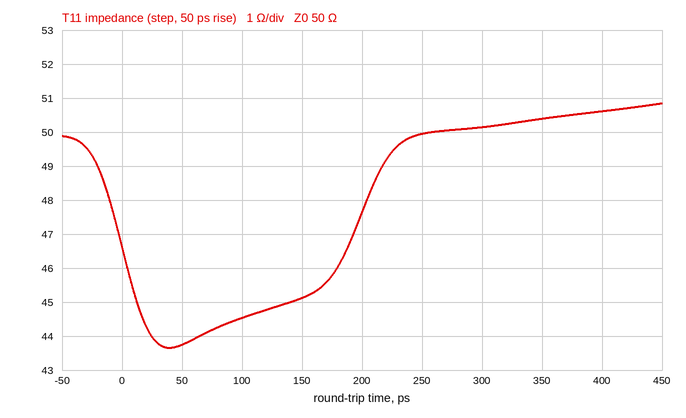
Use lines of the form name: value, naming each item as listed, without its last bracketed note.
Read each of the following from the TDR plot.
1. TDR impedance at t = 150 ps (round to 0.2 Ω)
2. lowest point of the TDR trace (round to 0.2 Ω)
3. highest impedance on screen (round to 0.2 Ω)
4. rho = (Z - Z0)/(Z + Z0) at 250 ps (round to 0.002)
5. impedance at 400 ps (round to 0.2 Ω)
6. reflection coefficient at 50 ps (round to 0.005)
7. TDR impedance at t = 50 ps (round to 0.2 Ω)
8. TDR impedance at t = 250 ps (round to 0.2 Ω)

TDR impedance at t = 150 ps: 45.2 Ω
lowest point of the TDR trace: 43.6 Ω
highest impedance on screen: 50.8 Ω
rho = (Z - Z0)/(Z + Z0) at 250 ps: 0.000
impedance at 400 ps: 50.6 Ω
reflection coefficient at 50 ps: -0.065
TDR impedance at t = 50 ps: 43.8 Ω
TDR impedance at t = 250 ps: 50.0 Ω
